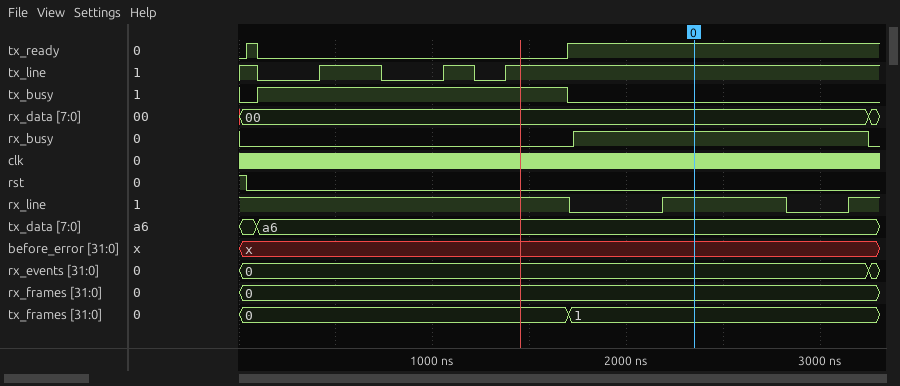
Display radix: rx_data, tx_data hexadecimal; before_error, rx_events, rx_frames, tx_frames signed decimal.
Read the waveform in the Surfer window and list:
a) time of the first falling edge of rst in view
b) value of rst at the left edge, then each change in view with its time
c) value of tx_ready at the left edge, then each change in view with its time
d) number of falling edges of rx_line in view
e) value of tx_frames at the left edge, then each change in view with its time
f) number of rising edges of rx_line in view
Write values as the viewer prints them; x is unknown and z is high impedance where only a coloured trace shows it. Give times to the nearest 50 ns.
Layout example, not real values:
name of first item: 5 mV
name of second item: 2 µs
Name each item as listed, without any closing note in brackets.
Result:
time of the first falling edge of rst in view: 50 ns
value of rst at the left edge, then each change in view with its time: 1, 0 at 50 ns
value of tx_ready at the left edge, then each change in view with its time: 0, 1 at 50 ns, 0 at 100 ns, 1 at 1700 ns
number of falling edges of rx_line in view: 2
value of tx_frames at the left edge, then each change in view with its time: 0, 1 at 1700 ns
number of rising edges of rx_line in view: 2
